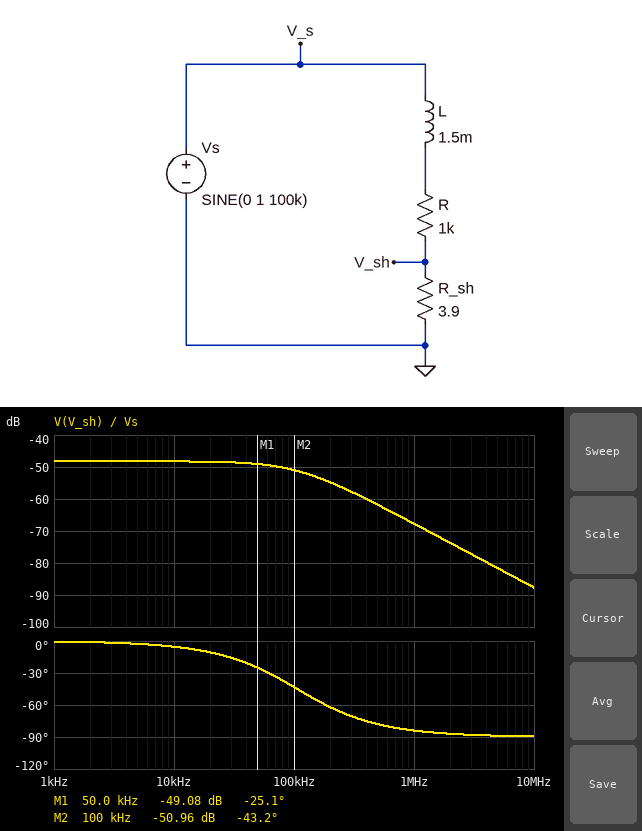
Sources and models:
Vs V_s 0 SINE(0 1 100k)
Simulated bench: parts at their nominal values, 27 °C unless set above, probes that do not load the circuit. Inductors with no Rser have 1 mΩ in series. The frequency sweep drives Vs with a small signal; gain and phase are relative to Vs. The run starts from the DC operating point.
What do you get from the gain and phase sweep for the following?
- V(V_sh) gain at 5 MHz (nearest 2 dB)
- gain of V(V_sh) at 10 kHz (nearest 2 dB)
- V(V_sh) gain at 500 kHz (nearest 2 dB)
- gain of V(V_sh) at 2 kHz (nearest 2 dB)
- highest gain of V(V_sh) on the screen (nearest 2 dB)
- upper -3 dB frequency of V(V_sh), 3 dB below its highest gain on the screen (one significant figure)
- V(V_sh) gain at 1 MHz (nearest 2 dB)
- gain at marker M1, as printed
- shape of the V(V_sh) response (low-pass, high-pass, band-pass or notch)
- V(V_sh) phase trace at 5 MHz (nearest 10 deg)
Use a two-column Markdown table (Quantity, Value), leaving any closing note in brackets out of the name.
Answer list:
| Quantity | Value |
|---|---|
| V(V_sh) gain at 5 MHz | -82 dB |
| gain of V(V_sh) at 10 kHz | -48 dB |
| V(V_sh) gain at 500 kHz | -62 dB |
| gain of V(V_sh) at 2 kHz | -48 dB |
| highest gain of V(V_sh) on the screen | -48 dB |
| upper -3 dB frequency of V(V_sh), 3 dB below its highest gain on the screen | 100 kHz |
| V(V_sh) gain at 1 MHz | -68 dB |
| gain at marker M1, as printed | -49.08 dB |
| shape of the V(V_sh) response | low-pass |
| V(V_sh) phase trace at 5 MHz | -90 deg |
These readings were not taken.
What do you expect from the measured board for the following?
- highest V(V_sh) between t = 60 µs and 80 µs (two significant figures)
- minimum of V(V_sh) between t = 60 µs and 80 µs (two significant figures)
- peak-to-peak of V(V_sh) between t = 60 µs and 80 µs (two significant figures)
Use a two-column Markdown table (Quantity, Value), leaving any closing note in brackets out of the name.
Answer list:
| Quantity | Value |
|---|---|
| highest V(V_sh) between t = 60 µs and 80 µs | 2.8 mV |
| minimum of V(V_sh) between t = 60 µs and 80 µs | -2.8 mV |
| peak-to-peak of V(V_sh) between t = 60 µs and 80 µs | 5.7 mV |
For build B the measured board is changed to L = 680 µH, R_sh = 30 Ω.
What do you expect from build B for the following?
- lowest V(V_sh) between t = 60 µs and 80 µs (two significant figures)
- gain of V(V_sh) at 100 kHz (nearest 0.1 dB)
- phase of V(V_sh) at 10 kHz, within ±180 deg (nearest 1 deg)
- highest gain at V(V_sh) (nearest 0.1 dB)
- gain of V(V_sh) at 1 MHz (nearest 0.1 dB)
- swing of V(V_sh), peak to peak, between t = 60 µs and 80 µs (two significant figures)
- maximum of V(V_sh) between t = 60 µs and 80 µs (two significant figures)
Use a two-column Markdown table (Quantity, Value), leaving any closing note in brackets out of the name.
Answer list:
| Quantity | Value |
|---|---|
| lowest V(V_sh) between t = 60 µs and 80 µs | -27 mV |
| gain of V(V_sh) at 100 kHz | -31.4 dB |
| phase of V(V_sh) at 10 kHz, within ±180 deg | -2 deg |
| highest gain at V(V_sh) | -30.7 dB |
| gain of V(V_sh) at 1 MHz | -43.3 dB |
| swing of V(V_sh), peak to peak, between t = 60 µs and 80 µs | 54 mV |
| maximum of V(V_sh) between t = 60 µs and 80 µs | 27 mV |
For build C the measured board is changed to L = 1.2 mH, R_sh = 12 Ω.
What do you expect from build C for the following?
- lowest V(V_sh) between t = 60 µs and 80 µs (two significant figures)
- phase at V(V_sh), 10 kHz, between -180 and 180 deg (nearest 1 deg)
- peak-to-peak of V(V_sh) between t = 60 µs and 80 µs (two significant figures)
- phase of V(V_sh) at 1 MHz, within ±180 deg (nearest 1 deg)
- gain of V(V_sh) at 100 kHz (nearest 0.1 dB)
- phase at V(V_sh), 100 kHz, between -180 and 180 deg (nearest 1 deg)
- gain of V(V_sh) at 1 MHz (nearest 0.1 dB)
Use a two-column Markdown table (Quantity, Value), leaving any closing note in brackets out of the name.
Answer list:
| Quantity | Value |
|---|---|
| lowest V(V_sh) between t = 60 µs and 80 µs | -9.5 mV |
| phase at V(V_sh), 10 kHz, between -180 and 180 deg | -4 deg |
| peak-to-peak of V(V_sh) between t = 60 µs and 80 µs | 19 mV |
| phase of V(V_sh) at 1 MHz, within ±180 deg | -82 deg |
| gain of V(V_sh) at 100 kHz | -40.4 dB |
| phase at V(V_sh), 100 kHz, between -180 and 180 deg | -37 deg |
| gain of V(V_sh) at 1 MHz | -56.0 dB |
